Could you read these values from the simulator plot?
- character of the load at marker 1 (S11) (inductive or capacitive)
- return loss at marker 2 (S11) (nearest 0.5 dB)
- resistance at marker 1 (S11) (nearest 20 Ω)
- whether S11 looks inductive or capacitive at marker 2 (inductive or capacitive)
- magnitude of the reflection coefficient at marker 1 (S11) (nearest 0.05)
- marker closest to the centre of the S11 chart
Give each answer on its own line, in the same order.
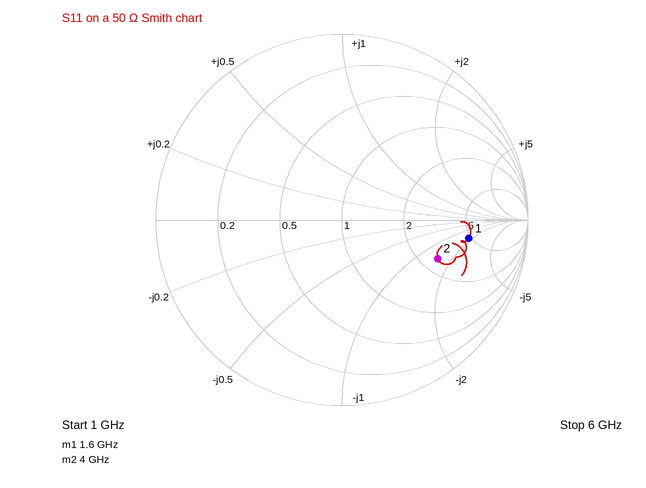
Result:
capacitive
5.0 dB
240 Ω
capacitive
0.70
marker 2
